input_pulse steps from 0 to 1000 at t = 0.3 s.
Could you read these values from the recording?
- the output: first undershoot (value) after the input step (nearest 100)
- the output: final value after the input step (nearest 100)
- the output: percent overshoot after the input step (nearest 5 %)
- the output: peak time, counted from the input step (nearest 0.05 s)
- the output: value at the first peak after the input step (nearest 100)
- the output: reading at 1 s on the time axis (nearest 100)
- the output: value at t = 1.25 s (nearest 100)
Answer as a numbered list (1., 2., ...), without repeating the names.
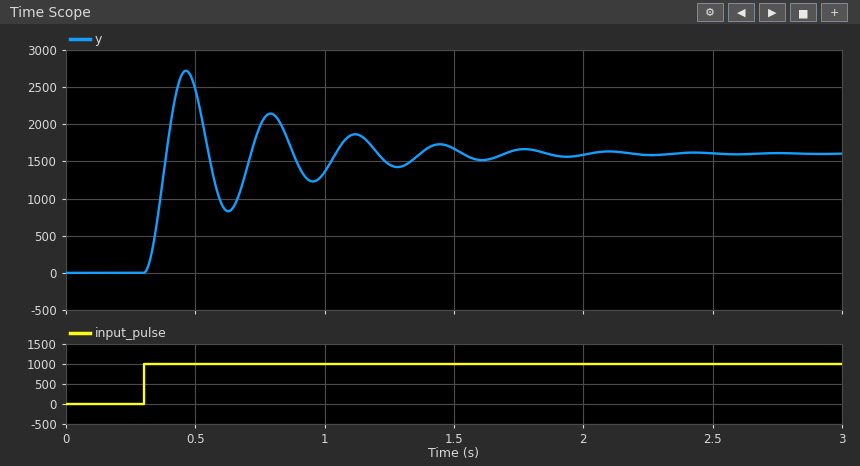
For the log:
1. 800
2. 1600
3. 70 %
4. 0.15 s
5. 2700
6. 1400
7. 1500
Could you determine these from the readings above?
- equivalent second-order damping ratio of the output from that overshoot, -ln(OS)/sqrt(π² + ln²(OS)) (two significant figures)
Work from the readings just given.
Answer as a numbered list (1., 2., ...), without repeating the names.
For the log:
1. 0.11
